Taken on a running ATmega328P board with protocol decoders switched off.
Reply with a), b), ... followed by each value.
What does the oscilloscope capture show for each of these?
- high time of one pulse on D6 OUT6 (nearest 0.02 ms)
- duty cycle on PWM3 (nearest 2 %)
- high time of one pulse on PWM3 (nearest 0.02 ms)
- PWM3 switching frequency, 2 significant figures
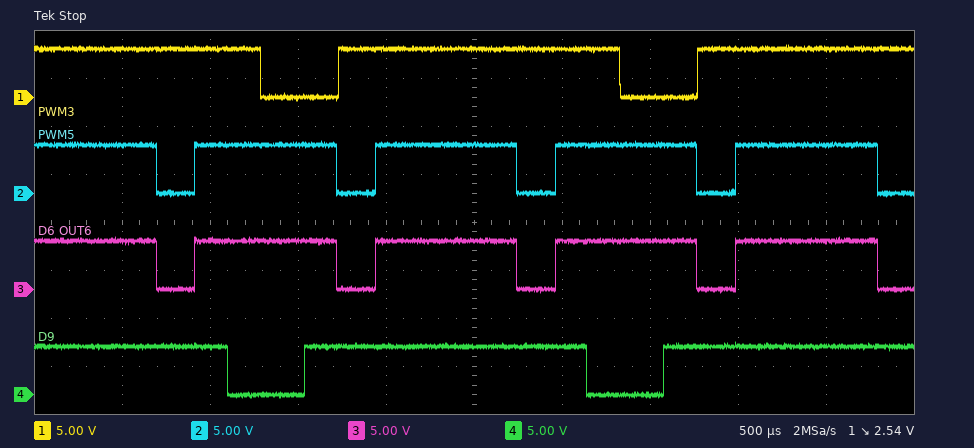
a) 0.80 ms
b) 78 %
c) 1.60 ms
d) 490 Hz
